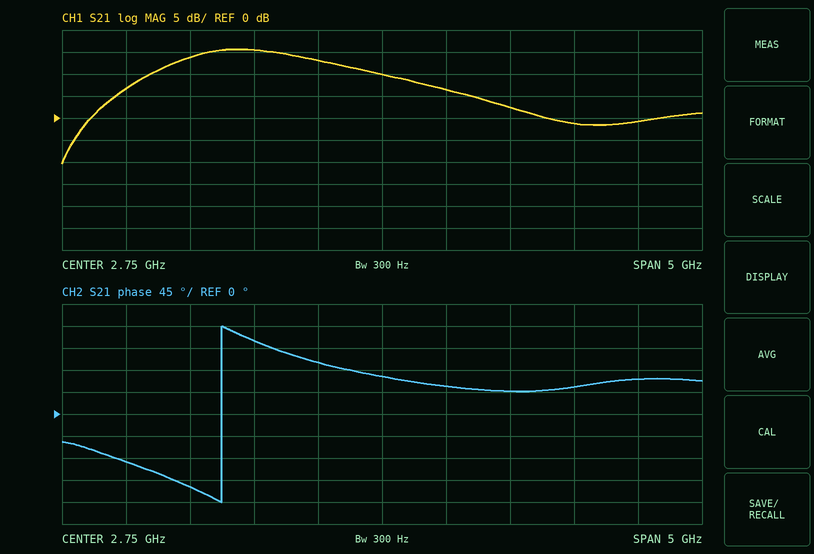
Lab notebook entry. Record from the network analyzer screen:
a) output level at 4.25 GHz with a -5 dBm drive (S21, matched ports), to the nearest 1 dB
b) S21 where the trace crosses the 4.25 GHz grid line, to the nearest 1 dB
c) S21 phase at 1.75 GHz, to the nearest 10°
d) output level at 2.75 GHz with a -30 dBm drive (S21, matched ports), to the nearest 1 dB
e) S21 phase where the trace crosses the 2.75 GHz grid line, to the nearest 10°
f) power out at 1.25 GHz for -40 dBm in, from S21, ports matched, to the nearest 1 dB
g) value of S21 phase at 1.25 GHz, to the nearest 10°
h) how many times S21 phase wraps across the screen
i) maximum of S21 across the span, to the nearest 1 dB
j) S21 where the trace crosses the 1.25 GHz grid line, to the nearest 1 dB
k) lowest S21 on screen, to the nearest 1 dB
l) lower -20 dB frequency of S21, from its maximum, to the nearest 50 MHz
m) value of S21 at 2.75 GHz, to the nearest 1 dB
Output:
-6 dBm
-1 dB
150°
-20 dBm
80°
-26 dBm
-150°
1
16 dB
14 dB
-10 dB
350 MHz
10 dB
